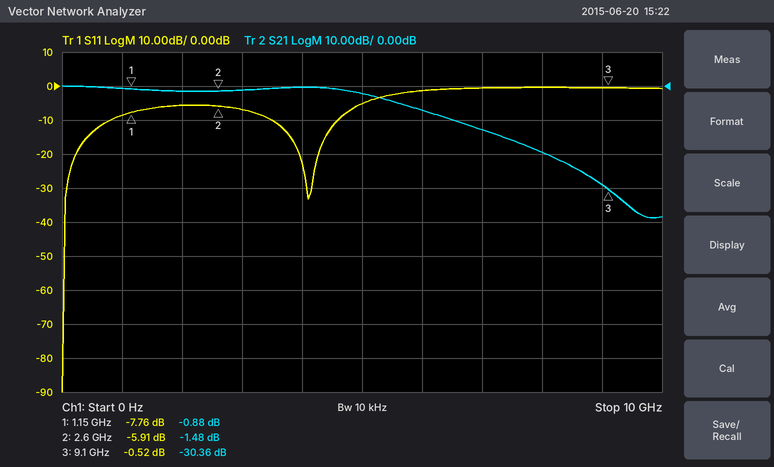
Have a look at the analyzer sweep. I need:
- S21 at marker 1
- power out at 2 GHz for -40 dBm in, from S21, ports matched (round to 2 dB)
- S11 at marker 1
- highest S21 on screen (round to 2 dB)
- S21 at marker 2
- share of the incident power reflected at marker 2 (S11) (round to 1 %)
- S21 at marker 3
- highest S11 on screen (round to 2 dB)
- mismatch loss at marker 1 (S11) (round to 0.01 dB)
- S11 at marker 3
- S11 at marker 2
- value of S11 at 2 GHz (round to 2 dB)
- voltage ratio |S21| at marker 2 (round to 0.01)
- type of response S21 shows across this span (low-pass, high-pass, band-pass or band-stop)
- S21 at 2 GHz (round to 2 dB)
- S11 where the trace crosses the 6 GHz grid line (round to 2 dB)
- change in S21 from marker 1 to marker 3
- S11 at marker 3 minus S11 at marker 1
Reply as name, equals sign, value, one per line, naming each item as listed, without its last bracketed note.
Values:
S21 at marker 1 = -0.88 dB
power out at 2 GHz for -40 dBm in, from S21, ports matched = -42 dBm
S11 at marker 1 = -7.76 dB
highest S21 on screen = 0 dB
S21 at marker 2 = -1.48 dB
share of the incident power reflected at marker 2 (S11) = 26 %
S21 at marker 3 = -30.36 dB
highest S11 on screen = 0 dB
mismatch loss at marker 1 (S11) = 0.80 dB
S11 at marker 3 = -0.52 dB
S11 at marker 2 = -5.91 dB
value of S11 at 2 GHz = -6 dB
voltage ratio |S21| at marker 2 = 0.84
type of response S21 shows across this span = low-pass
S21 at 2 GHz = -2 dB
S11 where the trace crosses the 6 GHz grid line = -2 dB
change in S21 from marker 1 to marker 3 = -29.48 dB
S11 at marker 3 minus S11 at marker 1 = 7.24 dB
